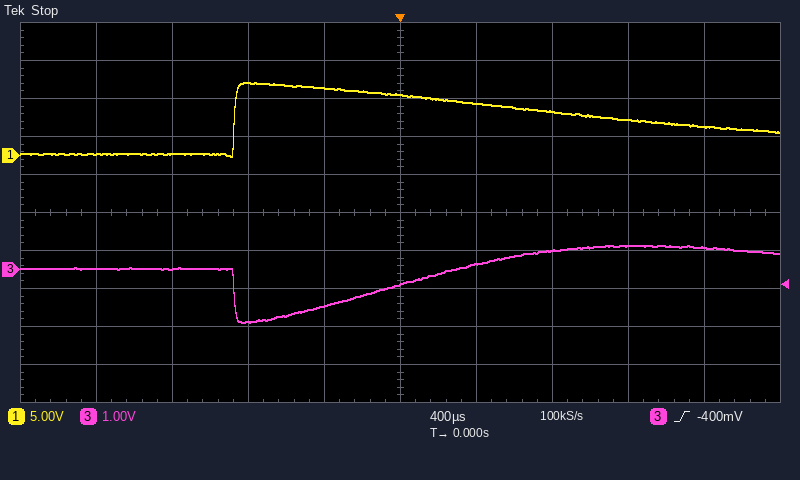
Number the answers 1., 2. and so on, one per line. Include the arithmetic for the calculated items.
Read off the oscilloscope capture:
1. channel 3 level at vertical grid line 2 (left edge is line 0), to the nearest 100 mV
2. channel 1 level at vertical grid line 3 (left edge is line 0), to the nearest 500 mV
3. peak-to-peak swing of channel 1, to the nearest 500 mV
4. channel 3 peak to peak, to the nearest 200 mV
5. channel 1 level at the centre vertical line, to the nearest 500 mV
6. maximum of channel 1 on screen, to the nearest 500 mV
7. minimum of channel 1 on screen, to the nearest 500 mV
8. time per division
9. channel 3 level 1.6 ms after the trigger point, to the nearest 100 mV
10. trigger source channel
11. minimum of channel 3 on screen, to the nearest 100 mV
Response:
1. 0.0 V
2. 9.5 V
3. 9.5 V − (0.0 V) = 9.5 V
4. 2.0 V
5. 8.0 V
6. 9.5 V
7. 0.0 V
8. 400 µs
9. 600 mV
10. channel 3
11. -1.4 V
